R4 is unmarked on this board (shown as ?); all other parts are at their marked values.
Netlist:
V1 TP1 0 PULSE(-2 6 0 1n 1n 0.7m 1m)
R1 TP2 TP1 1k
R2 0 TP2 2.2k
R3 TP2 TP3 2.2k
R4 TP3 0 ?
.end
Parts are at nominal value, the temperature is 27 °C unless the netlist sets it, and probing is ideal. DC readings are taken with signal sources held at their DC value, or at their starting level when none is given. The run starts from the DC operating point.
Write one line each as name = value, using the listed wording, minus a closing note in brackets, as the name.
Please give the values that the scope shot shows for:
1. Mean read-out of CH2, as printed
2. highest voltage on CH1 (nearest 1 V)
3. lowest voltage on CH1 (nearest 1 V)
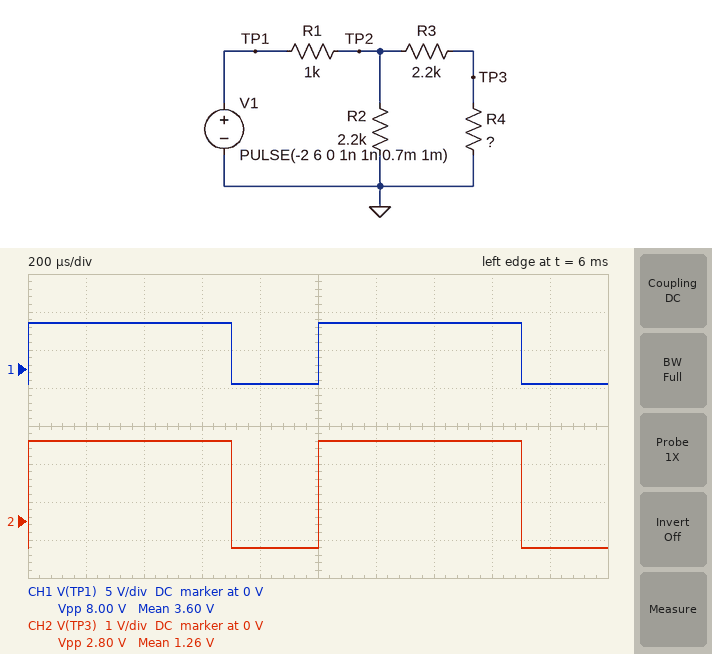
Mean read-out of CH2, as printed = 1.26 V
highest voltage on CH1 = 6 V
lowest voltage on CH1 = -2 V
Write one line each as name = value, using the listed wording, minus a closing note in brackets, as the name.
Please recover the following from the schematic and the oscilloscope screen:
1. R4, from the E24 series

R4, from the E24 series = 3 kΩ
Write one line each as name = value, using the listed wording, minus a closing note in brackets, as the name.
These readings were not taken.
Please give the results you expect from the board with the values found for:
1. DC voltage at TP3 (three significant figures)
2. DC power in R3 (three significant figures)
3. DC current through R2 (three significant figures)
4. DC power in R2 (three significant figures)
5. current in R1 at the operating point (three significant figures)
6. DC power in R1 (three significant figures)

DC voltage at TP3 = -701 mV
DC power in R3 = 120 µW
DC current through R2 = 552 µA
DC power in R2 = 670 µW
current in R1 at the operating point = 786 µA
DC power in R1 = 617 µW
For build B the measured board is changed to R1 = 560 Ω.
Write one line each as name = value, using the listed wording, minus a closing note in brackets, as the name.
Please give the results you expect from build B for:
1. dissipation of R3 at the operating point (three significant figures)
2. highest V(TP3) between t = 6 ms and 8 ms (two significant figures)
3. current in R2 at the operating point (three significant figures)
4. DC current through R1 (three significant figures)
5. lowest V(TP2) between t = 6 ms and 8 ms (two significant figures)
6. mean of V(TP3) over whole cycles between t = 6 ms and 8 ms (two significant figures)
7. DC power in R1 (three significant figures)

dissipation of R3 at the operating point = 175 µW
highest V(TP3) between t = 6 ms and 8 ms = 2.5 V
current in R2 at the operating point = 667 µA
DC current through R1 = 950 µA
lowest V(TP2) between t = 6 ms and 8 ms = -1.5 V
mean of V(TP3) over whole cycles between t = 6 ms and 8 ms = 1.5 V
DC power in R1 = 505 µW
